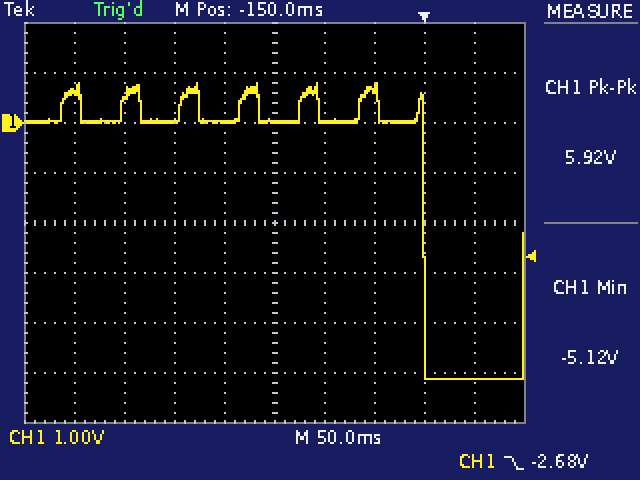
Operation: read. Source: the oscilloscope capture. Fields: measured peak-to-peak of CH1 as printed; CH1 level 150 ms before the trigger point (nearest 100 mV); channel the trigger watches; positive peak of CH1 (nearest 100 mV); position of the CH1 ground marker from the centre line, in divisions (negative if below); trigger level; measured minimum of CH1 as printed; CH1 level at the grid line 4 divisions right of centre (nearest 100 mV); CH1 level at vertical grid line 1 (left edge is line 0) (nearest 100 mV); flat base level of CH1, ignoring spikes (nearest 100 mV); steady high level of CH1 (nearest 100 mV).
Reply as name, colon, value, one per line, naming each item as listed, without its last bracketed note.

measured peak-to-peak of CH1 as printed: 5.92 V
CH1 level 150 ms before the trigger point: 0.0 V
channel the trigger watches: CH1
positive peak of CH1: 800 mV
position of the CH1 ground marker from the centre line, in divisions: +2.0 div
trigger level: -2.68 V
measured minimum of CH1 as printed: -5.12 V
CH1 level at the grid line 4 divisions right of centre: -5.1 V
CH1 level at vertical grid line 1 (left edge is line 0): 700 mV
flat base level of CH1, ignoring spikes: -5.1 V
steady high level of CH1: 0.0 V
